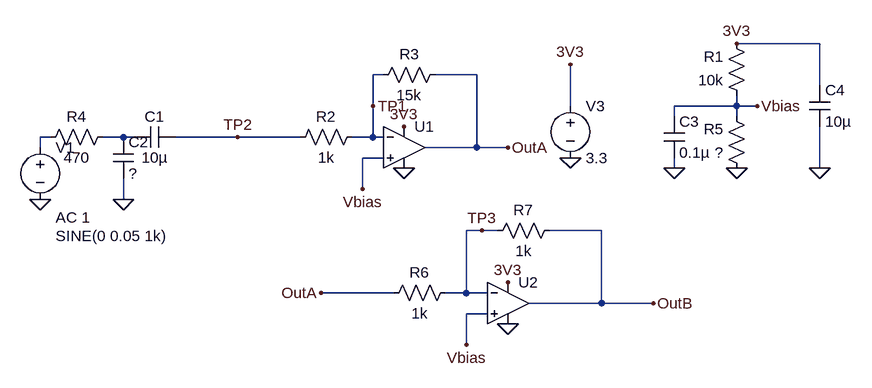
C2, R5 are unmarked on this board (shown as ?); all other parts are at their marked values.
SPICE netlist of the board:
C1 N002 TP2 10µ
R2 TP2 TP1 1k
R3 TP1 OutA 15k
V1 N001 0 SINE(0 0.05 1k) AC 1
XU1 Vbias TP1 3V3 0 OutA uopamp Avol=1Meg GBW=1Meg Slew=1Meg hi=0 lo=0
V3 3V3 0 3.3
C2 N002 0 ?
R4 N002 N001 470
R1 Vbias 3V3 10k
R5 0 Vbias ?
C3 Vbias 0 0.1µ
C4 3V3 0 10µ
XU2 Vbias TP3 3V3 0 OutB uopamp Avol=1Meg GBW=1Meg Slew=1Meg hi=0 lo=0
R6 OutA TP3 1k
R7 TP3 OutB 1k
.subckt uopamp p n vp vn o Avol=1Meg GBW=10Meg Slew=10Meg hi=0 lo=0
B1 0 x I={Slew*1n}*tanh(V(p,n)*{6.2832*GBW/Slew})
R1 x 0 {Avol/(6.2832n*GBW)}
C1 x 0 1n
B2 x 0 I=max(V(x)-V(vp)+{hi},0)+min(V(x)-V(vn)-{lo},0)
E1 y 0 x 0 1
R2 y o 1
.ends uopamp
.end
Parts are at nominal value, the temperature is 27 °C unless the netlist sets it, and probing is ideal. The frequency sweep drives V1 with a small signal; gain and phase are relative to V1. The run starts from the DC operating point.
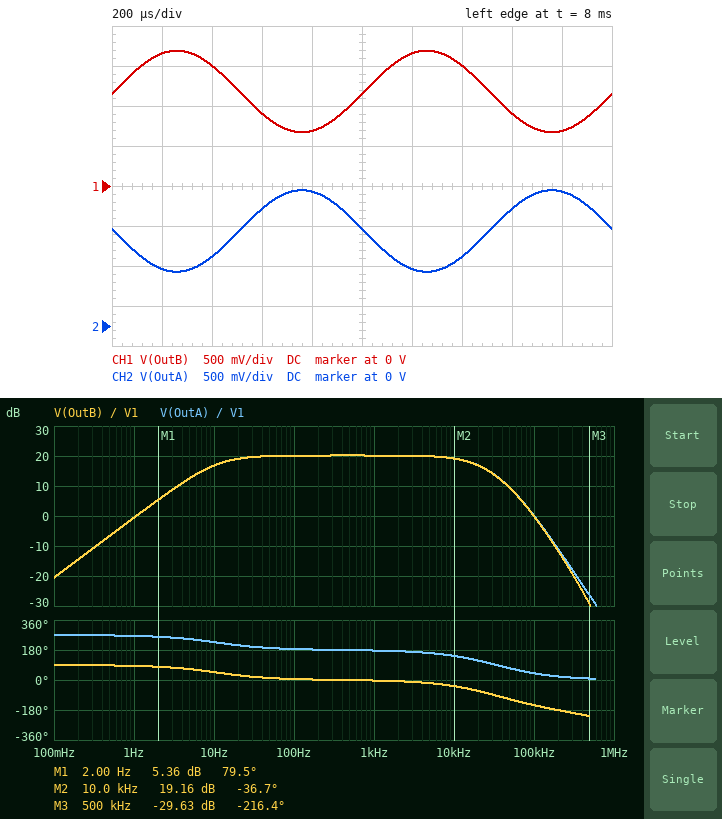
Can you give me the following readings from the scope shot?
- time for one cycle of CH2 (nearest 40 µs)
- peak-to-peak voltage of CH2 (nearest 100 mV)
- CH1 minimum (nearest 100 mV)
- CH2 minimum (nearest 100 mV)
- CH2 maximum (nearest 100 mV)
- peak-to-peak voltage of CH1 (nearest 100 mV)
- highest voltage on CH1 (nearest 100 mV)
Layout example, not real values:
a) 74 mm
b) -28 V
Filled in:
a) 1.00 ms
b) 1.0 V
c) 700 mV
d) 700 mV
e) 1.7 V
f) 1.0 V
g) 1.7 V
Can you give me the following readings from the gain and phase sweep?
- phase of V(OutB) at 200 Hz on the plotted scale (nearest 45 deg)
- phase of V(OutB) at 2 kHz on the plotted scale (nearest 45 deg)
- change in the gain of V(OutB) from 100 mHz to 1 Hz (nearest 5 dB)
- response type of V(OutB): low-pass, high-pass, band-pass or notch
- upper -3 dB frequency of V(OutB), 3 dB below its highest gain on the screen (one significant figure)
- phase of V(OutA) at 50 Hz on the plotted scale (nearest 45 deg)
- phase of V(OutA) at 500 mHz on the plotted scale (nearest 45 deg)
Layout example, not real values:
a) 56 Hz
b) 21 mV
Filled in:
a) 0 deg
b) 0 deg
c) 20 dB
d) band-pass
e) 20 kHz
f) 180 deg
g) 270 deg
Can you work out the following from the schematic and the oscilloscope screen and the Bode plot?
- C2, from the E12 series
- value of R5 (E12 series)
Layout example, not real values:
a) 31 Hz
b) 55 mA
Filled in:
a) 27 nF
b) 5.6 kΩ
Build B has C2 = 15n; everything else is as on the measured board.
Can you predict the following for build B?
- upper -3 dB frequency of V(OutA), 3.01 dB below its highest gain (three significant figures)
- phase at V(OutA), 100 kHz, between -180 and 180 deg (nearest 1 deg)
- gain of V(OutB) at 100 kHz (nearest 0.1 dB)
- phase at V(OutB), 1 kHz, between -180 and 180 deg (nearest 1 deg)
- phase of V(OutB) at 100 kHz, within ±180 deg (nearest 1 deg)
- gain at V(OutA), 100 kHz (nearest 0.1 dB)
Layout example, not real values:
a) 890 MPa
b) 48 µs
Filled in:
a) 31.9 kHz
b) 47 deg
c) 5.0 dB
d) -2 deg
e) -144 deg
f) 5.2 dB
